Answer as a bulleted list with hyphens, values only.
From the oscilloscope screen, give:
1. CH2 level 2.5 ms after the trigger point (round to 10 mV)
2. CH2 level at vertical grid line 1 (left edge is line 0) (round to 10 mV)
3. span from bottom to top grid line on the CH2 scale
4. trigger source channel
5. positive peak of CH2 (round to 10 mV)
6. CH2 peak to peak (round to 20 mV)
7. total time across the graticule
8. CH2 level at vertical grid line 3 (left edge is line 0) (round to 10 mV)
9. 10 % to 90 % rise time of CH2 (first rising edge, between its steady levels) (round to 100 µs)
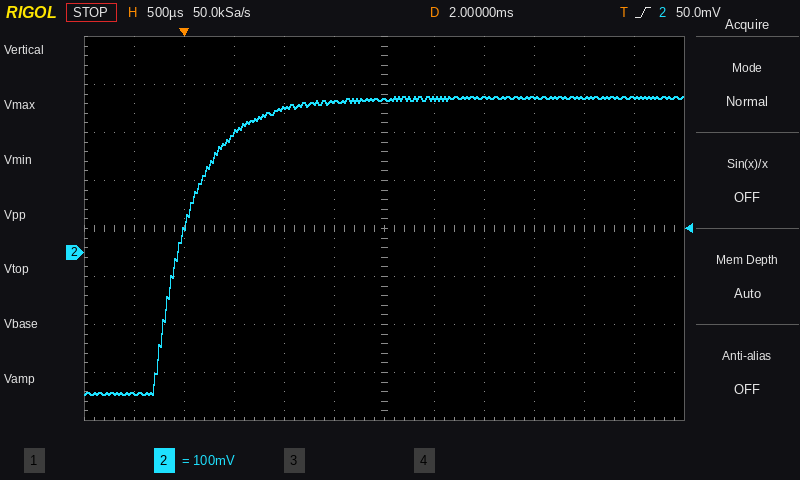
- 320 mV
- -290 mV
- 800 mV
- CH2
- 320 mV
- 620 mV
- 6 ms
- 250 mV
- 800 µs
